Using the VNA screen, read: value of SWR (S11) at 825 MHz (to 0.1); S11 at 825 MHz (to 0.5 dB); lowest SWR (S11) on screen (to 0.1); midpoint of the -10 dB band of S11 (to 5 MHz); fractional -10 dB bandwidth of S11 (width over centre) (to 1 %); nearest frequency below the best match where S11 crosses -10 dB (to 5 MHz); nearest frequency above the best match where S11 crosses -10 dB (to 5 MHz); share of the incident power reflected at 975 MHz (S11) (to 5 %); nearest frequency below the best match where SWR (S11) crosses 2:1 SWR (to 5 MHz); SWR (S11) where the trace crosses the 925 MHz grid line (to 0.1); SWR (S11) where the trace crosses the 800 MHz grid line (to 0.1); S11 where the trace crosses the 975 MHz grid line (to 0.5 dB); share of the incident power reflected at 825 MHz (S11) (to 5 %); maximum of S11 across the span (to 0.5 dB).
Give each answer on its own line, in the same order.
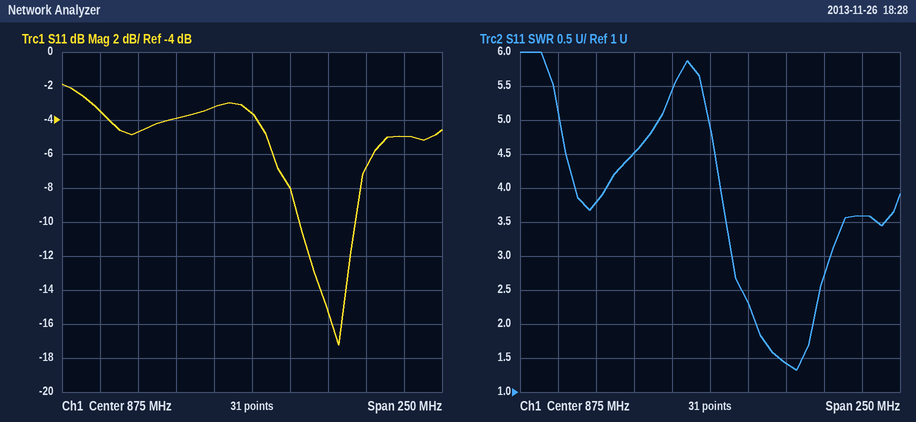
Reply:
4.5
-4.0 dB
1.3
925 MHz
4 %
905 MHz
945 MHz
30 %
905 MHz
1.4
3.8
-5.0 dB
40 %
-2.0 dB
